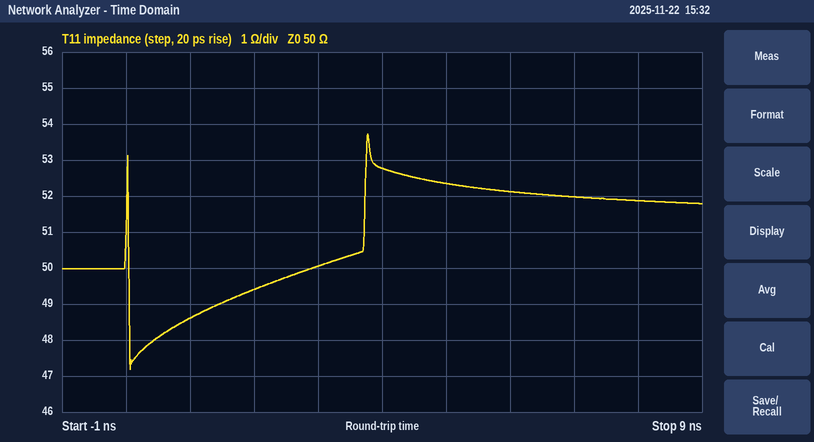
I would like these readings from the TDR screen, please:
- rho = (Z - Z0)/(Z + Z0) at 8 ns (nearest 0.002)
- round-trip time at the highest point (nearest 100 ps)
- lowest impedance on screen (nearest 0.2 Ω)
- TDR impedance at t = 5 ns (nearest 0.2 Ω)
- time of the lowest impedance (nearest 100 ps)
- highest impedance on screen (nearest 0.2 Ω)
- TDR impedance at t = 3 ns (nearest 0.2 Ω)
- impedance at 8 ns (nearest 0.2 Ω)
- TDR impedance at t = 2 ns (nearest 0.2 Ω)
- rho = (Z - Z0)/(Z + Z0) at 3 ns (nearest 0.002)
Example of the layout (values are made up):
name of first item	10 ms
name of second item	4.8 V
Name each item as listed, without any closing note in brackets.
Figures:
rho = (Z - Z0)/(Z + Z0) at 8 ns	+0.018
round-trip time at the highest point	3.8 ns
lowest impedance on screen	47.2 Ω
TDR impedance at t = 5 ns	52.4 Ω
time of the lowest impedance	100 ps
highest impedance on screen	53.8 Ω
TDR impedance at t = 3 ns	50.0 Ω
impedance at 8 ns	51.8 Ω
TDR impedance at t = 2 ns	49.4 Ω
rho = (Z - Z0)/(Z + Z0) at 3 ns	0.000
